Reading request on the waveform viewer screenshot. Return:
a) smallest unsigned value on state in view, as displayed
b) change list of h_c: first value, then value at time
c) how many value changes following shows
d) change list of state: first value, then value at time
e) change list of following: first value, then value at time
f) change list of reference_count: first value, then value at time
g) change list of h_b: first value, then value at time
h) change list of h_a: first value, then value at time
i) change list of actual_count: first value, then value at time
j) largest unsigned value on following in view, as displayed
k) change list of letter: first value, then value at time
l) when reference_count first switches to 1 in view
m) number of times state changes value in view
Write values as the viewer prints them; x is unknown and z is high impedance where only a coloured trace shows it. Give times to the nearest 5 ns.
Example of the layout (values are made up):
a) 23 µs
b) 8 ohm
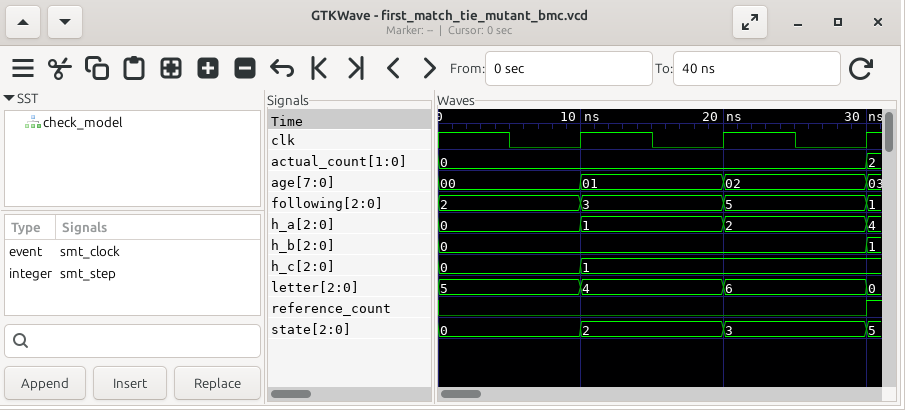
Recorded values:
a) 0
b) 0, 1 at 10 ns
c) 3
d) 0, 2 at 10 ns, 3 at 20 ns, 5 at 30 ns
e) 2, 3 at 10 ns, 5 at 20 ns, 1 at 30 ns
f) 0, 1 at 30 ns
g) 0, 1 at 30 ns
h) 0, 1 at 10 ns, 2 at 20 ns, 4 at 30 ns
i) 0, 2 at 30 ns
j) 5
k) 5, 4 at 10 ns, 6 at 20 ns, 0 at 30 ns
l) 30 ns
m) 3
